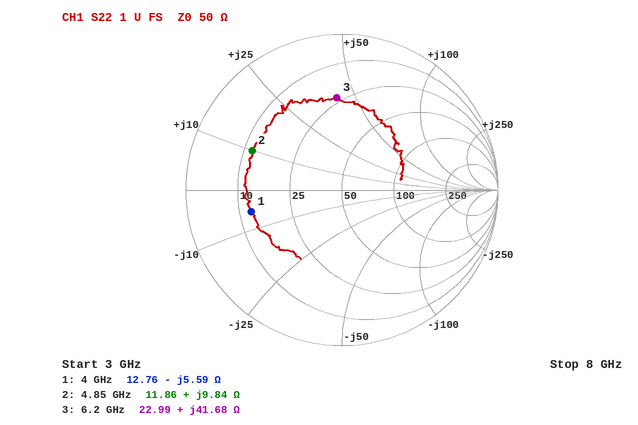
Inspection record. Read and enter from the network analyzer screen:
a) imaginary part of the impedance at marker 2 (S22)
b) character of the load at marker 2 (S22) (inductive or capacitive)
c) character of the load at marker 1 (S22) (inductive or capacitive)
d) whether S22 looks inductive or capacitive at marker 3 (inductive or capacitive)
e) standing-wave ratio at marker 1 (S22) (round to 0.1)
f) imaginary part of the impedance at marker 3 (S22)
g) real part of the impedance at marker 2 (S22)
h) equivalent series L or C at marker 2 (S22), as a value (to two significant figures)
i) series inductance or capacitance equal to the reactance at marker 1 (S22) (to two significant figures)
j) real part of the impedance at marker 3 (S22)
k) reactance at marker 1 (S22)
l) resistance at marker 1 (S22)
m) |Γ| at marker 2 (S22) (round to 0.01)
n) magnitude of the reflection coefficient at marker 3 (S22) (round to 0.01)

+9.84 Ω
inductive
capacitive
inductive
4.0
+41.68 Ω
11.86 Ω
320 pH
7.1 pF
22.99 Ω
-5.59 Ω
12.76 Ω
0.63
0.59
